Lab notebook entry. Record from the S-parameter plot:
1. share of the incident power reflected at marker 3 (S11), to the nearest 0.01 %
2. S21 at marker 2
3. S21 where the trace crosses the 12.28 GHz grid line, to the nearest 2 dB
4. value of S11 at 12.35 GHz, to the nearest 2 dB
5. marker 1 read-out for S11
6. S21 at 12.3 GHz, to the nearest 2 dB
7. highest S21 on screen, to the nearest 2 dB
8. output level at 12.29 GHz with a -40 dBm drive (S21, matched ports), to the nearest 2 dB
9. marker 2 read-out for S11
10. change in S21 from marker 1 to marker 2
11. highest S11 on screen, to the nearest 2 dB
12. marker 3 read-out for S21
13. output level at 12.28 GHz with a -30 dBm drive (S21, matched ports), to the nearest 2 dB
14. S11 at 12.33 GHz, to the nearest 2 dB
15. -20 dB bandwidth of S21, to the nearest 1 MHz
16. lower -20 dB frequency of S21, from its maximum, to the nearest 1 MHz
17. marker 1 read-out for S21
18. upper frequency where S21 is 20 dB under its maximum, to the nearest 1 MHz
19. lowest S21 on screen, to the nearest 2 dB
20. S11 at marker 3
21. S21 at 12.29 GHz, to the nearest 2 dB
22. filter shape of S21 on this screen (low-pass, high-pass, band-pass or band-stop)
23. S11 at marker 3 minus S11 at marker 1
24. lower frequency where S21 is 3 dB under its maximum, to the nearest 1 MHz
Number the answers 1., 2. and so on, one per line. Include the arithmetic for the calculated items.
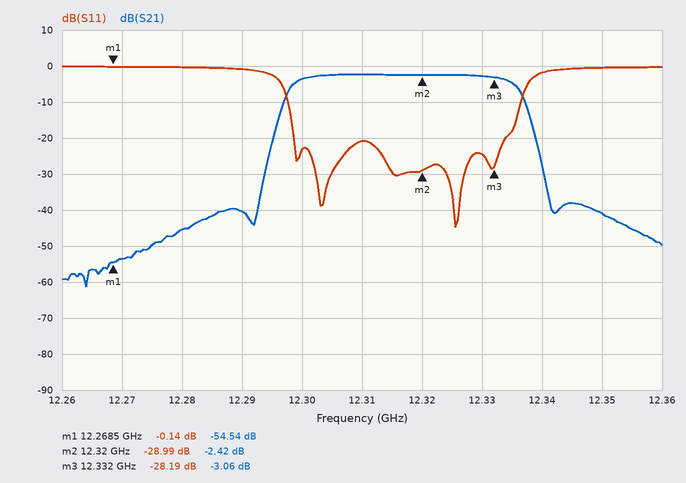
1. 10^(-28.19/10) ≈ 0.15 %
2. -2.42 dB
3. -46 dB
4. 0 dB
5. -0.14 dB
6. -4 dB
7. -2 dB
8. -40 dBm + (-40 dB) = -80 dBm
9. -28.99 dB
10. -2.42 − (-54.54) = 52.12 dB
11. 0 dB
12. -3.06 dB
13. -30 dBm + (-46 dB) = -76 dBm
14. -24 dB
15. 12.339 GHz − 12.295 GHz = 44 MHz
16. 12.295 GHz
17. -54.54 dB
18. 12.339 GHz
19. -62 dB
20. -28.19 dB
21. -40 dB
22. band-pass
23. -28.19 − (-0.14) = -28.05 dB
24. 12.298 GHz
